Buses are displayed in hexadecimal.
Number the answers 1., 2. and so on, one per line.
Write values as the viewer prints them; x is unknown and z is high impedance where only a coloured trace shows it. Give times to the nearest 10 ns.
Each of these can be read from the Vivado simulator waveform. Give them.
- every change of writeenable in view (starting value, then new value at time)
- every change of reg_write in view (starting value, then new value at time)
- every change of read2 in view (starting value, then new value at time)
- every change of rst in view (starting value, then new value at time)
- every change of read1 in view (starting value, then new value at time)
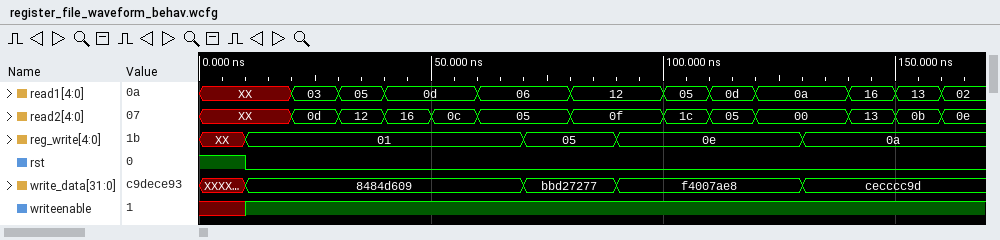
1. x, 1 at 10 ns
2. XX, 01 at 10 ns, 05 at 70 ns, 0e at 90 ns, 0a at 130 ns
3. XX, 0d at 20 ns, 12 at 30 ns, 16 at 40 ns, 0c at 50 ns, 05 at 60 ns, 0f at 80 ns, 1c at 100 ns, 05 at 110 ns, 00 at 120 ns, 13 at 140 ns, 0b at 150 ns, 0e at 160 ns
4. 1, 0 at 10 ns
5. XX, 03 at 20 ns, 05 at 30 ns, 0d at 40 ns, 06 at 60 ns, 12 at 80 ns, 05 at 100 ns, 0d at 110 ns, 0a at 120 ns, 16 at 140 ns, 13 at 150 ns, 02 at 160 ns
